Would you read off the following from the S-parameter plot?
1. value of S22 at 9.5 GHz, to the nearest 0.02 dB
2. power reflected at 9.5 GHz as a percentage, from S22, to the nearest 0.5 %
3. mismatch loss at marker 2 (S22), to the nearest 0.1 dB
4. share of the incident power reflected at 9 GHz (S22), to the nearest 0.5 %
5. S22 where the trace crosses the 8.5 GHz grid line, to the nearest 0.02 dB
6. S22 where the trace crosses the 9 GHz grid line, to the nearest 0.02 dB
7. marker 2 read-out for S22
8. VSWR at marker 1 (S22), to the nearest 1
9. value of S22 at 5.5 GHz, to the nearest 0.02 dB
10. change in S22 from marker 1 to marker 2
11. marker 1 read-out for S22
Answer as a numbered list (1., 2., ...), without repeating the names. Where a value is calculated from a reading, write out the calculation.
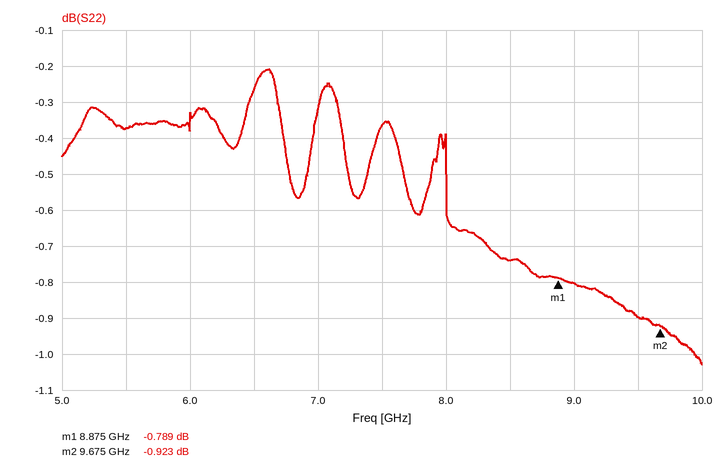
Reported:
1. -0.90 dB
2. 10^(-0.9/10) ≈ 81.3 %, so 81.5 % to the nearest 0.5 %
3. −10 log10(1 − 10^(-0.923/10)) ≈ 7.2 dB
4. 10^(-0.8/10) ≈ 83.2 %, so 83.0 % to the nearest 0.5 %
5. -0.74 dB
6. -0.80 dB
7. -0.923 dB
8. (1 + 0.9132)/(1 − 0.9132) ≈ 22
9. -0.38 dB
10. -0.923 − (-0.789) = -0.134 dB
11. -0.789 dB
